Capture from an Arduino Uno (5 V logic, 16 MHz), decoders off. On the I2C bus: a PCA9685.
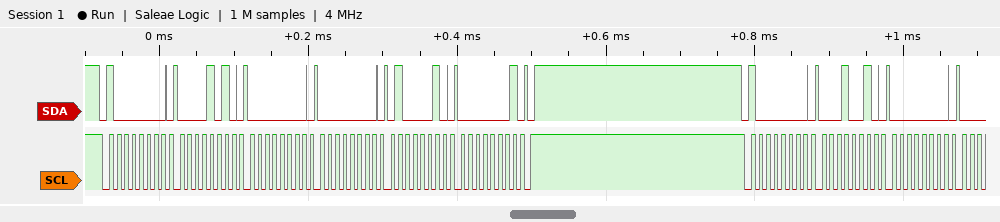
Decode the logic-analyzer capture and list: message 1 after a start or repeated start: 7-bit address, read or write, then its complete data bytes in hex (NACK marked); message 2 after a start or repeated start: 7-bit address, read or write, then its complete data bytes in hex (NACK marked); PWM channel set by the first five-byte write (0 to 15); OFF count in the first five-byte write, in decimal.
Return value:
0x40 write: 0A 00 00 42 01
0x40 write: 12 00
1
322
